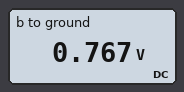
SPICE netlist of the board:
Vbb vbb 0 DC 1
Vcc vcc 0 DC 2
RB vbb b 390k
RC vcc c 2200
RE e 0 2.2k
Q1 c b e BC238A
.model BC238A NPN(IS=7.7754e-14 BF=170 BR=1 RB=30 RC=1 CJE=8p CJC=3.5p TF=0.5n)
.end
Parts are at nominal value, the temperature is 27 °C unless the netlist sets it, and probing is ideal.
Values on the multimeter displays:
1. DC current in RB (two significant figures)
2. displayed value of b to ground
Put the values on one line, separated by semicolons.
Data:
600 nA; 0.767 V
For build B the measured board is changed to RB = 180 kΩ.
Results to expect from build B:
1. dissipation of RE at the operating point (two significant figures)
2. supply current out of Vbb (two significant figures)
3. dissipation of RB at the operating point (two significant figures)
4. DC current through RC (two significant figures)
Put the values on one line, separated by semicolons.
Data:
42 µW; 810 nA; 120 nW; 140 µA
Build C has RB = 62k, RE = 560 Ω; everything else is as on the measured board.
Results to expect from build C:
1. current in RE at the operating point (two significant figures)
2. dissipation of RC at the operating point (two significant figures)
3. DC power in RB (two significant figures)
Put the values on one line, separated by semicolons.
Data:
450 µA; 450 µW; 440 nW
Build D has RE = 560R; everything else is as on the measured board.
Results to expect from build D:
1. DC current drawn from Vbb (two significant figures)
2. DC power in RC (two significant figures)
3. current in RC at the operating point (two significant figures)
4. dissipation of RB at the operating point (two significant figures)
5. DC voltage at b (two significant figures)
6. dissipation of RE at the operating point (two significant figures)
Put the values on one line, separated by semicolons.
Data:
920 nA; 54 µW; 160 µA; 330 nW; 640 mV; 14 µW
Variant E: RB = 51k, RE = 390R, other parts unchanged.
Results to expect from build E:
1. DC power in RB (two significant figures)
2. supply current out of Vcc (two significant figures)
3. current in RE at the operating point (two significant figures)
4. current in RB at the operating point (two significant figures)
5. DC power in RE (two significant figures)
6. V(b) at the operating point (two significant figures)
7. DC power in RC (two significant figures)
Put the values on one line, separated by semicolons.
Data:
620 nW; 590 µA; 600 µA; 3.5 µA; 140 µW; 820 mV; 780 µW
